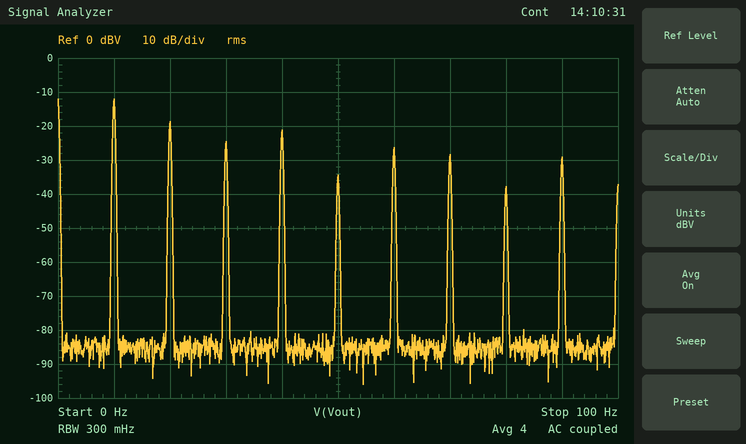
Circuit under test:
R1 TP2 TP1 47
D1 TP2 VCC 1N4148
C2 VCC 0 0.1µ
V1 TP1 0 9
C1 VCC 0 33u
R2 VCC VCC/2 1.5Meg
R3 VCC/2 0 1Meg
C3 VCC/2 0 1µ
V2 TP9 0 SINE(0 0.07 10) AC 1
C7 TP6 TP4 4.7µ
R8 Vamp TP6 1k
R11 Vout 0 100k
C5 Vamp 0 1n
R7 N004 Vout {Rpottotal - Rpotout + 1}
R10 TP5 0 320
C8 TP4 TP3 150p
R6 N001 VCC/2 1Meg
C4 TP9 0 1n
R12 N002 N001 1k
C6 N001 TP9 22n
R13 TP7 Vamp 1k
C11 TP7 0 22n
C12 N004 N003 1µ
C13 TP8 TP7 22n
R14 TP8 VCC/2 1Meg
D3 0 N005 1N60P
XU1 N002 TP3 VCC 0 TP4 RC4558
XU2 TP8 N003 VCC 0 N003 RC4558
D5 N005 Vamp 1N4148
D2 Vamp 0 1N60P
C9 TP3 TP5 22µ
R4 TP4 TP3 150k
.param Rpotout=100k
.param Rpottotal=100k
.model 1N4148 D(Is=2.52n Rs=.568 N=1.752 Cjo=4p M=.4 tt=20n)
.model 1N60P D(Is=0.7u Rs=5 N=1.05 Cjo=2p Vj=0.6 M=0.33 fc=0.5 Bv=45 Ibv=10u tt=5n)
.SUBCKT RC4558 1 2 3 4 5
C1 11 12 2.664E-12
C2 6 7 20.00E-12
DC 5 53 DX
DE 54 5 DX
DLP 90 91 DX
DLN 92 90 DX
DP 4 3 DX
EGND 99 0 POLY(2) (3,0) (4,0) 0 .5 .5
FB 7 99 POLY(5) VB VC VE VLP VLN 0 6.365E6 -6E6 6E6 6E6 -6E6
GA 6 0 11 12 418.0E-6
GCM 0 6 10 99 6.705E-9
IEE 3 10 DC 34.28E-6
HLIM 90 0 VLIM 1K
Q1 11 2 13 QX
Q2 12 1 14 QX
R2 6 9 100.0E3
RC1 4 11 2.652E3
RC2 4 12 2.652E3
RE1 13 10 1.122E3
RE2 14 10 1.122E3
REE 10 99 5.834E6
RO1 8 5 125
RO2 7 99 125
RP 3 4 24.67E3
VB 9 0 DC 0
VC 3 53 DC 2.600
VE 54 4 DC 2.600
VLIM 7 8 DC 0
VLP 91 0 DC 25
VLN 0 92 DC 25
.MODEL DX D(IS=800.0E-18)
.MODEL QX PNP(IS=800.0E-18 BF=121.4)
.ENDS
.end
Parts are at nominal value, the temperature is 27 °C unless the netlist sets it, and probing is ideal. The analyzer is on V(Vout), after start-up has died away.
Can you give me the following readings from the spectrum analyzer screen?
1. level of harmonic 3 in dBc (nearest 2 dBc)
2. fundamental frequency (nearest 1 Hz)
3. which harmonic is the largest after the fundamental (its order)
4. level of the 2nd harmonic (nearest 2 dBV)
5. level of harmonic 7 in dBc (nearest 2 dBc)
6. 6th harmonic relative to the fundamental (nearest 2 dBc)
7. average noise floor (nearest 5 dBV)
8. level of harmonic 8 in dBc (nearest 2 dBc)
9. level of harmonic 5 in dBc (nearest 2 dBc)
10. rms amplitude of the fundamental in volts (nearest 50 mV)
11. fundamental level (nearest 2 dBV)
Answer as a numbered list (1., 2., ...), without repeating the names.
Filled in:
1. -12 dBc
2. 10 Hz
3. 2
4. -18 dBV
5. -16 dBc
6. -14 dBc
7. -85 dBV
8. -26 dBc
9. -22 dBc
10. 250 mV
11. -12 dBV
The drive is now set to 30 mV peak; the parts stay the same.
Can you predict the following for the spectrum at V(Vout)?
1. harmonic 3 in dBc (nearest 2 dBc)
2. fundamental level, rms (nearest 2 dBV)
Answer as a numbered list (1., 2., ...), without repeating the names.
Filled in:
1. -14 dBc
2. -12 dBV
